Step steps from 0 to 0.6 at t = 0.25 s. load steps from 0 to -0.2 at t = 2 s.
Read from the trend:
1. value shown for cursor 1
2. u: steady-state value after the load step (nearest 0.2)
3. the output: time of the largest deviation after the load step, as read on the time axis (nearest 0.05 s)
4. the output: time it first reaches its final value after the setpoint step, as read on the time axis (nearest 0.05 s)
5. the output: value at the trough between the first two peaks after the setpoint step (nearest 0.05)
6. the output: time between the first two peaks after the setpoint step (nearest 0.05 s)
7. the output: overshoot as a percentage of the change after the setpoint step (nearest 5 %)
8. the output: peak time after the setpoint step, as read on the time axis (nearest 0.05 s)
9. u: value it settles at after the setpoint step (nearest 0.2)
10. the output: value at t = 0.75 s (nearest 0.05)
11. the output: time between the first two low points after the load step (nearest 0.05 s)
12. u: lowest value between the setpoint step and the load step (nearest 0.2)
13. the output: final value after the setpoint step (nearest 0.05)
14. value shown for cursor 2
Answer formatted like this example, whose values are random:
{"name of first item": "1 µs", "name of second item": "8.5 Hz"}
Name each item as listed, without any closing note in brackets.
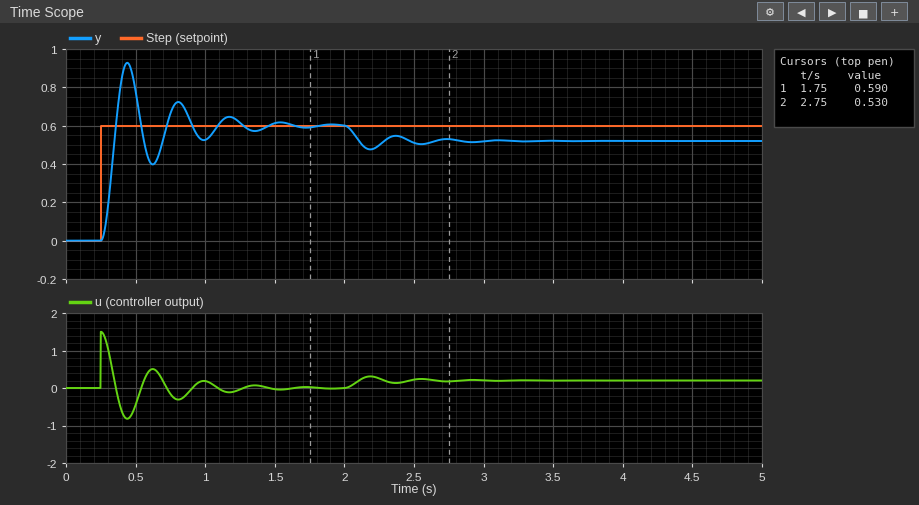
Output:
{"value shown for cursor 1": "0.590", "u: steady-state value after the load step": "0.2", "the output: time of the largest deviation after the load step, as read on the time axis": "2.20 s", "the output: time it first reaches its final value after the setpoint step, as read on the time axis": "0.35 s", "the output: value at the trough between the first two peaks after the setpoint step": "0.40", "the output: time between the first two peaks after the setpoint step": "0.35 s", "the output: overshoot as a percentage of the change after the setpoint step": "55 %", "the output: peak time after the setpoint step, as read on the time axis": "0.45 s", "u: value it settles at after the setpoint step": "0.0", "the output: value at t = 0.75 s": "0.65", "the output: time between the first two low points after the load step": "0.35 s", "u: lowest value between the setpoint step and the load step": "-0.8", "the output: final value after the setpoint step": "0.60", "value shown for cursor 2": "0.530"}
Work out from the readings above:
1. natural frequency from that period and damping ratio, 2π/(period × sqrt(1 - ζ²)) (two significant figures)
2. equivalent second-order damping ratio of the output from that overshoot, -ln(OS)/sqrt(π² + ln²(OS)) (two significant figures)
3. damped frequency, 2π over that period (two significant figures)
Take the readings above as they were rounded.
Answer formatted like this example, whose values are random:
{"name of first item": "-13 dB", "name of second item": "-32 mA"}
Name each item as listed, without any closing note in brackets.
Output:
{"natural frequency from that period and damping ratio, 2π/(period × sqrt(1 - ζ²))": "18 rad/s", "equivalent second-order damping ratio of the output from that overshoot, -ln(OS)/sqrt(π² + ln²(OS))": "0.19", "damped frequency, 2π over that period": "18 rad/s"}
